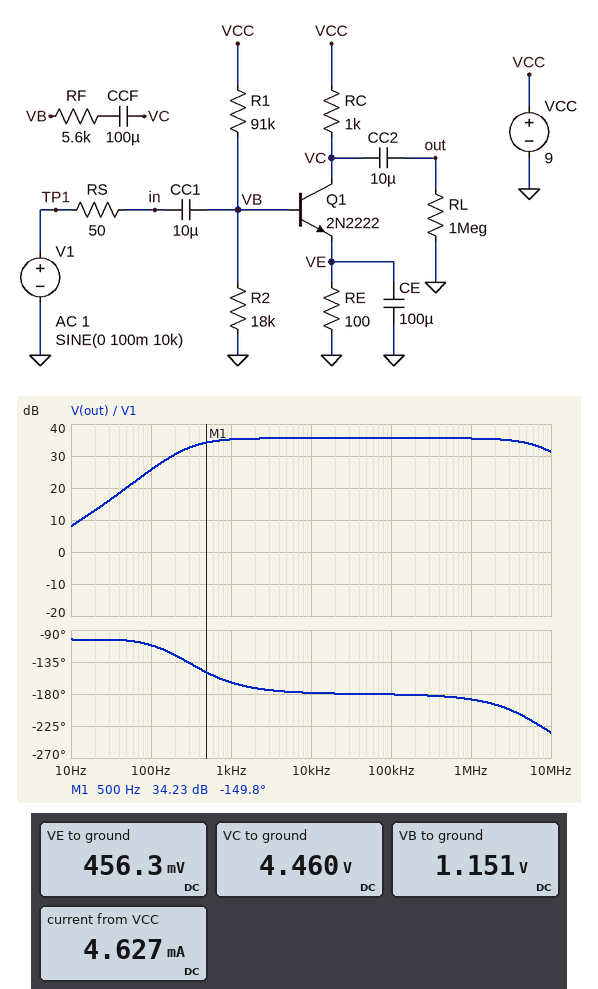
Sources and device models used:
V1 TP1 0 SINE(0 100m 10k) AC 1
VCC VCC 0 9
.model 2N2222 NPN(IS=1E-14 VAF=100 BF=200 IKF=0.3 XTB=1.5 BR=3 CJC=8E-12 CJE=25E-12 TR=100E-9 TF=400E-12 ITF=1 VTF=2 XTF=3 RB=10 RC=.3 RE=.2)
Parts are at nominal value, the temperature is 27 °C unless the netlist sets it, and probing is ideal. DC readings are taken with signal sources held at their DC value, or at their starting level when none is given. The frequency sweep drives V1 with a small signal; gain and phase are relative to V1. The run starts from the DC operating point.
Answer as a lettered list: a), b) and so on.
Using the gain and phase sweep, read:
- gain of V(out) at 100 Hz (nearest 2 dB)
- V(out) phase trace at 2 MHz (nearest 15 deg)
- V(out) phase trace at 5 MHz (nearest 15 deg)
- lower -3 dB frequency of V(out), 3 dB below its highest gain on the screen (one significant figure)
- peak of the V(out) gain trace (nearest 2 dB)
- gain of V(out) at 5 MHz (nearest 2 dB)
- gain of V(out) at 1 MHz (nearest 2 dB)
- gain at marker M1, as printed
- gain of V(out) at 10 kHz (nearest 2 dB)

a) 26 dB
b) -195 deg
c) -210 deg
d) 300 Hz
e) 36 dB
f) 34 dB
g) 36 dB
h) 34.23 dB
i) 36 dB
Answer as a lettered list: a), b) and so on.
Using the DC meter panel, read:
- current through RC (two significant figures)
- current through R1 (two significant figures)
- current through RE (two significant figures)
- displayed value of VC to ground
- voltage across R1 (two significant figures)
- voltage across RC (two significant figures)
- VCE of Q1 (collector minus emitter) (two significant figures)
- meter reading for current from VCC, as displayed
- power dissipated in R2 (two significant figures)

a) 4.5 mA
b) 86 µA
c) 4.6 mA
d) 4.460 V
e) 7.8 V
f) 4.5 V
g) 4.0 V
h) 4.627 mA
i) 74 µW
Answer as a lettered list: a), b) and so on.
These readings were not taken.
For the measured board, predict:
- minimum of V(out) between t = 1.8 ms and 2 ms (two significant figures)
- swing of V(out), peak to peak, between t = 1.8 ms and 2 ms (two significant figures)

a) -3.9 V
b) 7.6 V
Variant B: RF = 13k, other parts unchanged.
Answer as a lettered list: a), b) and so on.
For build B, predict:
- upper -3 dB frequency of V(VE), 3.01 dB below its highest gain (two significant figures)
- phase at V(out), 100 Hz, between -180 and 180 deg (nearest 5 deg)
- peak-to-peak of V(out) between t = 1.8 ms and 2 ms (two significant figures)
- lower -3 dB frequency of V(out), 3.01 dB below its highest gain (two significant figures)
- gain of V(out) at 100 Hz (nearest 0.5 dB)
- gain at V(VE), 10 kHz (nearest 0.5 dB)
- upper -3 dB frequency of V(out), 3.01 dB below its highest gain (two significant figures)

a) 300 Hz
b) -115 deg
c) 8.1 V
d) 290 Hz
e) 29.5 dB
f) -36.0 dB
g) 5.1 MHz
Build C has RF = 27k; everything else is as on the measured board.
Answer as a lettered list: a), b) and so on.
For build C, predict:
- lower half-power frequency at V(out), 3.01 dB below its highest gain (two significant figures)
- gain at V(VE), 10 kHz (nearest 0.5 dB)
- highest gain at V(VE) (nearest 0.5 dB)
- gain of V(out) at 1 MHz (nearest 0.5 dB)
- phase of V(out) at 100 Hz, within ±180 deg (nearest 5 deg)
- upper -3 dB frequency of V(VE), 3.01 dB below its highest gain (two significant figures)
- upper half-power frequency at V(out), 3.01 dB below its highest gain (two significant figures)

a) 280 Hz
b) -34.5 dB
c) -3.5 dB
d) 41.0 dB
e) -115 deg
f) 290 Hz
g) 4.0 MHz
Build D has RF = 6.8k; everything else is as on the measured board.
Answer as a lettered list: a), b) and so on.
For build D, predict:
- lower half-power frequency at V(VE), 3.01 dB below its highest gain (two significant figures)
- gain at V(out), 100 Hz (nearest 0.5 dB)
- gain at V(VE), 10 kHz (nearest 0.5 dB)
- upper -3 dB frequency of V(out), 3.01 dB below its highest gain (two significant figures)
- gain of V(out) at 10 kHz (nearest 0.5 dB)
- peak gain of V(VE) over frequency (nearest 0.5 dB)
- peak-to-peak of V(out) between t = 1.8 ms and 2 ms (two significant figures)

a) 9.6 Hz
b) 26.5 dB
c) -38.0 dB
d) 6.9 MHz
e) 36.5 dB
f) -8.0 dB
g) 7.7 V
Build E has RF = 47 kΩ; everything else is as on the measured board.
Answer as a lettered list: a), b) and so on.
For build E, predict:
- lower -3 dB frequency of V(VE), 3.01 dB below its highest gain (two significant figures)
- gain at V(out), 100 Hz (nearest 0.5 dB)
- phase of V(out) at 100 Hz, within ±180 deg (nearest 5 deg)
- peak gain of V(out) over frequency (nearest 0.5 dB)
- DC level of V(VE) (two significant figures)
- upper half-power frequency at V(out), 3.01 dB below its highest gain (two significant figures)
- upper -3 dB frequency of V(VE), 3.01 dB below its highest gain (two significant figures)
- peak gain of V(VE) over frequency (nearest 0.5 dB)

a) 4.1 Hz
b) 33.0 dB
c) -115 deg
d) 42.0 dB
e) 460 mV
f) 3.6 MHz
g) 290 Hz
h) -2.5 dB
